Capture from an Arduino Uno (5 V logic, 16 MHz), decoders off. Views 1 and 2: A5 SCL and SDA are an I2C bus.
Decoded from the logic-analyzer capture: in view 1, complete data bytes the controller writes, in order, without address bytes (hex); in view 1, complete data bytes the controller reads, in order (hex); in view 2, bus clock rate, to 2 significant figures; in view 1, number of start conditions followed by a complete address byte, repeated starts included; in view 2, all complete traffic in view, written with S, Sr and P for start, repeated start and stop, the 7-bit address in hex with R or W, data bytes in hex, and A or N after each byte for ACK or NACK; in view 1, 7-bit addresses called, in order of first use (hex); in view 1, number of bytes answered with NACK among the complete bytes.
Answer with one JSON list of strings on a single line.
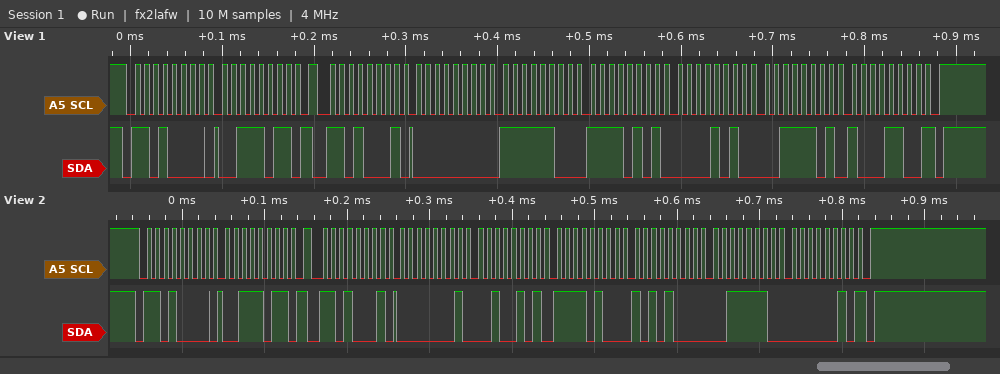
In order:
["3B", "00 FC F5 0A 3D 8C", "100 kHz", "2", "S 68W A 3B A Sr 68R A 01 A 25 A F4 A A8 A 3E A 02 N P", "0x68", "1"]
